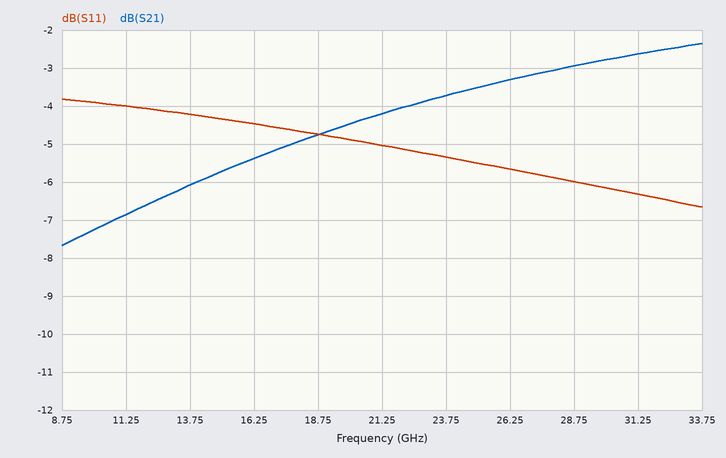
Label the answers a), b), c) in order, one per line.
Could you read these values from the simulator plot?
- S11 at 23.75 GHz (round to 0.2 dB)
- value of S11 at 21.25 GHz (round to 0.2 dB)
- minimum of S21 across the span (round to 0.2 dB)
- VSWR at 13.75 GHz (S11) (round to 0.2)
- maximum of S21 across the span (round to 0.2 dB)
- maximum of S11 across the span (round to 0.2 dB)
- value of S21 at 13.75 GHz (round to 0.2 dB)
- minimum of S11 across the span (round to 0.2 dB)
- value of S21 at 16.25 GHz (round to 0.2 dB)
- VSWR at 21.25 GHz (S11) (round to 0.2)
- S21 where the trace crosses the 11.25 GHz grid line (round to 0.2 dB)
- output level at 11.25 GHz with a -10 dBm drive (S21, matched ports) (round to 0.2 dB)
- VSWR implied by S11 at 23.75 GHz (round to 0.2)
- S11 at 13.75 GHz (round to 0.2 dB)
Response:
a) -5.4 dB
b) -5.0 dB
c) -7.6 dB
d) 4.2
e) -2.4 dB
f) -3.8 dB
g) -6.0 dB
h) -6.6 dB
i) -5.4 dB
j) 3.6
k) -6.8 dB
l) -16.8 dBm
m) 3.4
n) -4.2 dB
